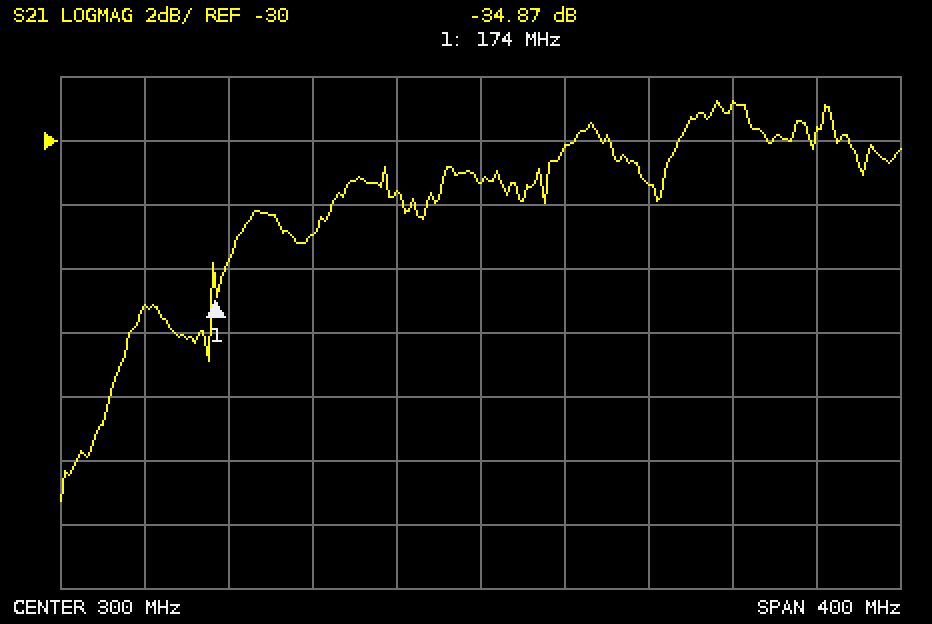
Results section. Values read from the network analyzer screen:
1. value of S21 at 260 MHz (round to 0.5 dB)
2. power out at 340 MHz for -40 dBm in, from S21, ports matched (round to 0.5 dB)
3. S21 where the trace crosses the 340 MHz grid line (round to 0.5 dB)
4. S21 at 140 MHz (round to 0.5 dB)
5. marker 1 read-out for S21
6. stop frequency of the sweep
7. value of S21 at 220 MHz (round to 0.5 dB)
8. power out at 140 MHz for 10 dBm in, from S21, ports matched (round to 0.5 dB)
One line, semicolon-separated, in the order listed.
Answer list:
-31.5 dB; -70.0 dBm; -30.0 dB; -35.0 dB; -34.87 dB; 500 MHz; -33.0 dB; -25.0 dBm
